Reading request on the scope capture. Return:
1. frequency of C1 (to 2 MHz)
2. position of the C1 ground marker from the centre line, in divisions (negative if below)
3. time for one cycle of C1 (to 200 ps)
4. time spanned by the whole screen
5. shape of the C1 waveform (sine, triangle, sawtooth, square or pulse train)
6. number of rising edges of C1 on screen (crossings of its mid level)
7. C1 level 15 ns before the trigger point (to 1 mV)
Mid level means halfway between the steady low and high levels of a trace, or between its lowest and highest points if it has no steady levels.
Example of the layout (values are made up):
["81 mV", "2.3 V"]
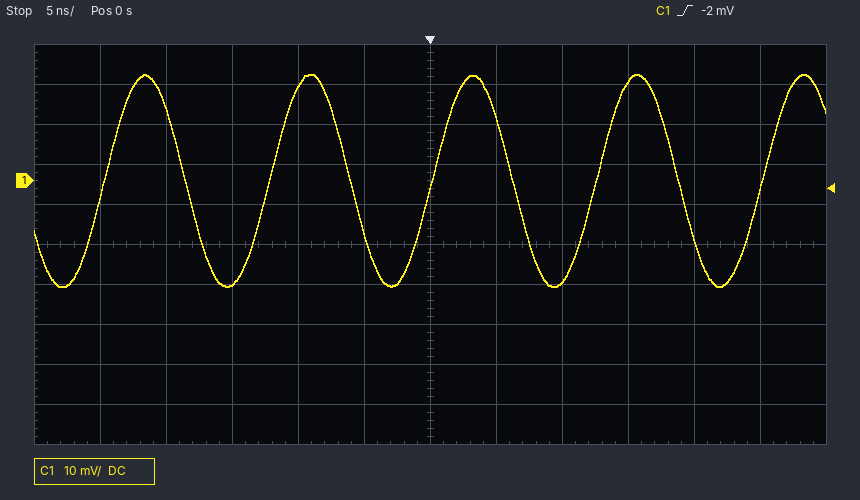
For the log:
["80 MHz", "+1.6 div", "12.4 ns", "60 ns", "sine", "5", "-26 mV"]
